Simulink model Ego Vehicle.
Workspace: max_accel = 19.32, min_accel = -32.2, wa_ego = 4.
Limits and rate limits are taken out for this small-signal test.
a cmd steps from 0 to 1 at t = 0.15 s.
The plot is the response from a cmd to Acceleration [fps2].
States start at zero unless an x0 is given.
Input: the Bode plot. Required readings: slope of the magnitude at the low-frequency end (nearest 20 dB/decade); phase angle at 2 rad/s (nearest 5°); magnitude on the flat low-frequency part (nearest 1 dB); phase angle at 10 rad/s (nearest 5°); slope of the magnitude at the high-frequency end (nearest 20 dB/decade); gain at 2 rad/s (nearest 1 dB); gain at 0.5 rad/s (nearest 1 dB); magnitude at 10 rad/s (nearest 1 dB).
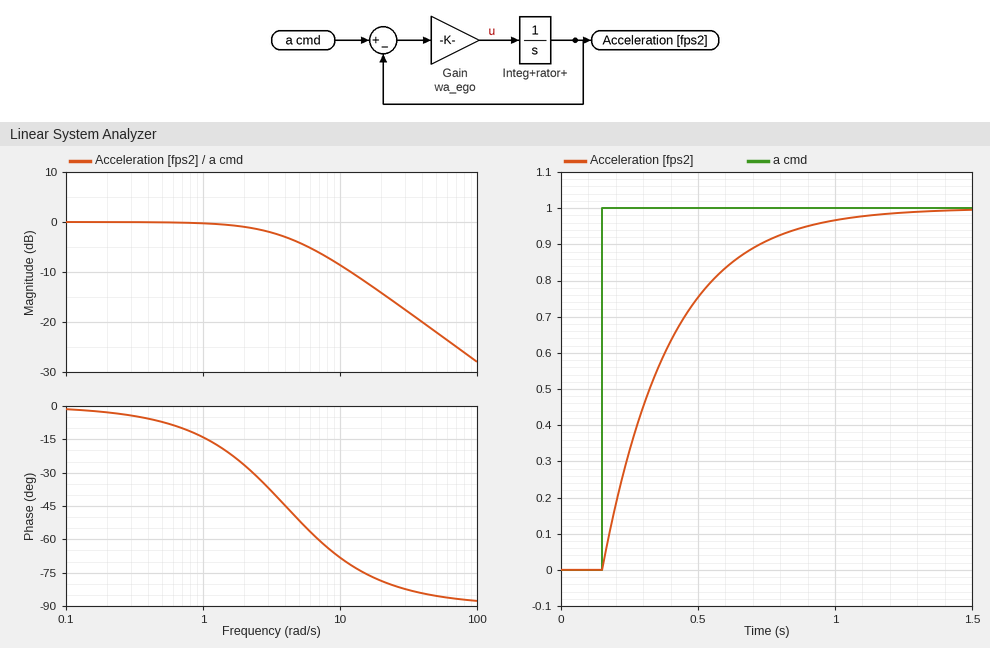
0 dB/decade
-25°
0 dB
-70°
-20 dB/decade
-1 dB
0 dB
-9 dB
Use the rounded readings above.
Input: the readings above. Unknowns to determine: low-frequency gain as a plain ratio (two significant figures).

1.0
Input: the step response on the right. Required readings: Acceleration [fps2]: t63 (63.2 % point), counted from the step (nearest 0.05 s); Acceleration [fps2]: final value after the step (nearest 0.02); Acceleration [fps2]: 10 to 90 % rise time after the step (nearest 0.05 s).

0.25 s
1.00
0.55 s
